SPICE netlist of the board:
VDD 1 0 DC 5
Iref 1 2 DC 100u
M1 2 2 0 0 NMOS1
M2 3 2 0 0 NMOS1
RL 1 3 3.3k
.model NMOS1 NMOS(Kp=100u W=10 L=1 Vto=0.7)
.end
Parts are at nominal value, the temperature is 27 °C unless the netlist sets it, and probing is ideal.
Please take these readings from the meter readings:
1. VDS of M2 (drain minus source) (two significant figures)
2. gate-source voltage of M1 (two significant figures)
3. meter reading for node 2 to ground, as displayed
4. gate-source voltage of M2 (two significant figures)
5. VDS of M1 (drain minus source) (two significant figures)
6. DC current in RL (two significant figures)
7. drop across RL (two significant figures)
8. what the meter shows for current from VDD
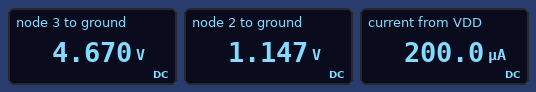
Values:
4.7 V
1.1 V
1.147 V
1.1 V
1.1 V
100 µA
330 mV
200.0 µA
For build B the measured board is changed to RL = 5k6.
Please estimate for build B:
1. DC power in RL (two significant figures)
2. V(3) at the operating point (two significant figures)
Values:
56 µW
4.4 V
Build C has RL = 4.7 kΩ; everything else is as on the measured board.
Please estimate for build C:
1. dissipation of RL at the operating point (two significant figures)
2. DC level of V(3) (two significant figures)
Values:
47 µW
4.5 V
